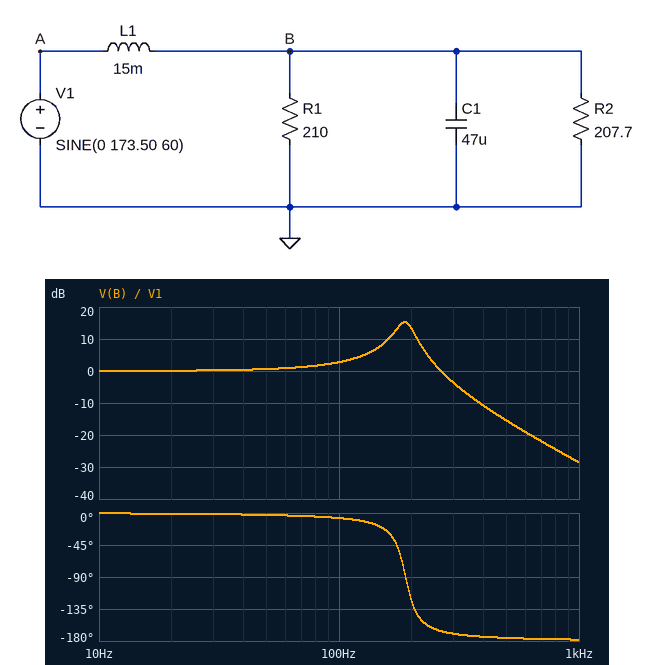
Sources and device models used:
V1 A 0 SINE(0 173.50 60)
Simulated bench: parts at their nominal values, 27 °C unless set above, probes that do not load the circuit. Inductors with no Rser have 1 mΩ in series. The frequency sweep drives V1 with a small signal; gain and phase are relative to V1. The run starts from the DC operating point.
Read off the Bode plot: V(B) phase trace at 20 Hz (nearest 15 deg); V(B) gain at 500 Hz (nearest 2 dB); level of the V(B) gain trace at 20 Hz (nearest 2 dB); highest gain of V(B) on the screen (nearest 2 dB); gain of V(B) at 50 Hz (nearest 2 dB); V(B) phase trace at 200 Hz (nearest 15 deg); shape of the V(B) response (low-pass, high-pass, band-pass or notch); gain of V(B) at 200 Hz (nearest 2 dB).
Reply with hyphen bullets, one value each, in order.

- 0 deg
- -16 dB
- 0 dB
- 16 dB
- 0 dB
- -120 deg
- low-pass
- 14 dB
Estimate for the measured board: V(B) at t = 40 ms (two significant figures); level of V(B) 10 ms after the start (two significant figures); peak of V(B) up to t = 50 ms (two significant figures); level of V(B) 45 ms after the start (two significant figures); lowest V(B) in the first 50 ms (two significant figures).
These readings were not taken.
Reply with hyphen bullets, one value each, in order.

- 120 V
- -86 V
- 230 V
- -180 V
- -210 V
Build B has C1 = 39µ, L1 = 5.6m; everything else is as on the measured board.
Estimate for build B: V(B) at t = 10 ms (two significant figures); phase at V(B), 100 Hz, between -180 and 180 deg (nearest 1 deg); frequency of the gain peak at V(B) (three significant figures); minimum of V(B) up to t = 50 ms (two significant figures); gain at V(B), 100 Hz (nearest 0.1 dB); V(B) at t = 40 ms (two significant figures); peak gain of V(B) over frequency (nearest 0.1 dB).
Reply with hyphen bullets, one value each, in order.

- -110 V
- -2 deg
- 339 Hz
- -190 V
- 0.8 dB
- 110 V
- 18.8 dB
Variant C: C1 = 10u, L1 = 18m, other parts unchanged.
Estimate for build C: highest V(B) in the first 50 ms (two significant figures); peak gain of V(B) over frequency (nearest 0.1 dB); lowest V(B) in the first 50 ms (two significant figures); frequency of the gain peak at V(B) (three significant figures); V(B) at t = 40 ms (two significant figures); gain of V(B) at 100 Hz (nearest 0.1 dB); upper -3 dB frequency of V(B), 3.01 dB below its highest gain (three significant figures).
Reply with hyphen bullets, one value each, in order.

- 180 V
- 8.0 dB
- -180 V
- 359 Hz
- 110 V
- 0.6 dB
- 430 Hz
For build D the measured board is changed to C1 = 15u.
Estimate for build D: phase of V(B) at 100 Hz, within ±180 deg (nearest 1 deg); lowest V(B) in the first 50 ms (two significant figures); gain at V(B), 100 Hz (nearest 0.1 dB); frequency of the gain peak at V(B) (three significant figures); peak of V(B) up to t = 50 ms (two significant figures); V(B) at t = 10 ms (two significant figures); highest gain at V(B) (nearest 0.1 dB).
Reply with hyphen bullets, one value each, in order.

- -6 deg
- -180 V
- 0.8 dB
- 328 Hz
- 180 V
- -98 V
- 10.5 dB
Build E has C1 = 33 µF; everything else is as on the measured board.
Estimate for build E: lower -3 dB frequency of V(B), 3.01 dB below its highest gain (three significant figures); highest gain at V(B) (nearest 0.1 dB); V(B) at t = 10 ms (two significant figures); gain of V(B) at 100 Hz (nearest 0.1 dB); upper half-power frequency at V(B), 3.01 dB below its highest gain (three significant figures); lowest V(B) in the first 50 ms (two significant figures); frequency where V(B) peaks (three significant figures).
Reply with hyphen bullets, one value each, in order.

- 199 Hz
- 13.8 dB
- -110 V
- 1.8 dB
- 246 Hz
- -190 V
- 224 Hz
